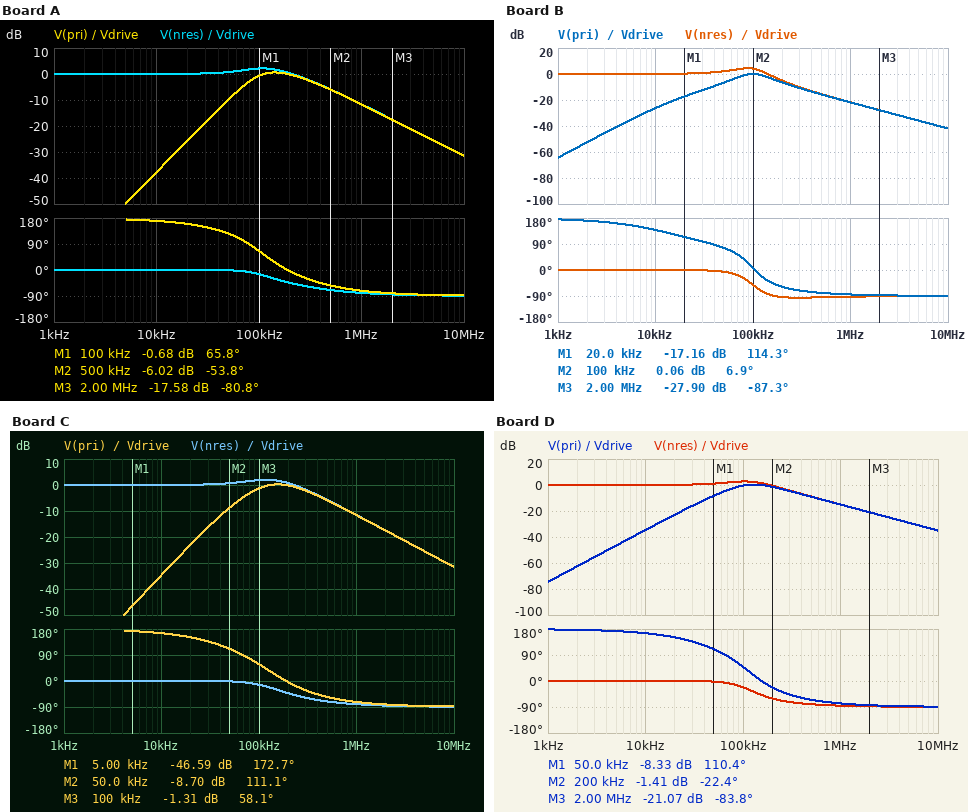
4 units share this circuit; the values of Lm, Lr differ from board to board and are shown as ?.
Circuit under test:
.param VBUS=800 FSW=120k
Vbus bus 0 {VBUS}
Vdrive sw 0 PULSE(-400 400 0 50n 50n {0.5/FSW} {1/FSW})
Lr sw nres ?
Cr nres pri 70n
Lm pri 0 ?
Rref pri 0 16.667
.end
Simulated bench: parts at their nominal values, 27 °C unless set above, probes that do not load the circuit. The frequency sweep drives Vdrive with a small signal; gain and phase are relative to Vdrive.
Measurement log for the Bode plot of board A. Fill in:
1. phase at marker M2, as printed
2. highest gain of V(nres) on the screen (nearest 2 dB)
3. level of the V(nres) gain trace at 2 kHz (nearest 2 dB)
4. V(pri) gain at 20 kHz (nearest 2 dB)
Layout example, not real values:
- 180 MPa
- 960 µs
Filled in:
- -53.8 deg
- 2 dB
- 0 dB
- -26 dB
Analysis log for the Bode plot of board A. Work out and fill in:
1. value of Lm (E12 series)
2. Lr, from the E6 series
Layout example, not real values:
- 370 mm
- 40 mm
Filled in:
- 47 µH
- 10 µH
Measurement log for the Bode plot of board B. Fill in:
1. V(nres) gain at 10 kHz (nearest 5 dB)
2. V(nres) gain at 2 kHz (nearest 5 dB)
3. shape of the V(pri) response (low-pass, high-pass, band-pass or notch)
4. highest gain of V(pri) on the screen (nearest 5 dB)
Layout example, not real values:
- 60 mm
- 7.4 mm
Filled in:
- 0 dB
- 0 dB
- band-pass
- 0 dB
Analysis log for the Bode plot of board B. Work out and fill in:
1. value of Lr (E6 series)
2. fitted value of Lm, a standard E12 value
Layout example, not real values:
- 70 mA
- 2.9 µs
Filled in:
- 33 µH
- 220 µH
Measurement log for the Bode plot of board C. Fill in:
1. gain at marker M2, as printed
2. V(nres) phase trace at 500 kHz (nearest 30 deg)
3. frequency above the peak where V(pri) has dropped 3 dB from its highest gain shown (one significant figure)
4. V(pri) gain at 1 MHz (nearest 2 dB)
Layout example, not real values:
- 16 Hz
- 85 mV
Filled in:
- -8.70 dB
- -60 deg
- 300 kHz
- -12 dB
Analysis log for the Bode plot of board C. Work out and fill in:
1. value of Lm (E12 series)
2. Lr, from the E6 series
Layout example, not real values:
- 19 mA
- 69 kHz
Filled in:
- 68 µH
- 10 µH
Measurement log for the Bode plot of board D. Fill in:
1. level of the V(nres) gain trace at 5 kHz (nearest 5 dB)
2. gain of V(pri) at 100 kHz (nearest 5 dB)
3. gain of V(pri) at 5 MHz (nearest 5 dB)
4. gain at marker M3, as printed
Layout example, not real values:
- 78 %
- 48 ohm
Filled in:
- 0 dB
- 0 dB
- -30 dB
- -21.07 dB
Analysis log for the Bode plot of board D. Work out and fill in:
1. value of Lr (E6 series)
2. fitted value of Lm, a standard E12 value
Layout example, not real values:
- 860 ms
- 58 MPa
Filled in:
- 15 µH
- 68 µH
